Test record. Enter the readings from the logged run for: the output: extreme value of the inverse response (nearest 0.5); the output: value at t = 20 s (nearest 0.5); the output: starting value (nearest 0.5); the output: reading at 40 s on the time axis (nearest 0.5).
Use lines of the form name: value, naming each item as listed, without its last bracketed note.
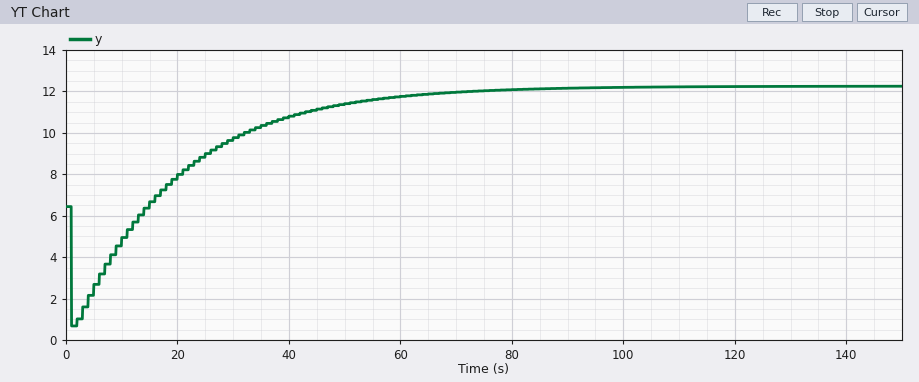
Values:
the output: extreme value of the inverse response: 0.5
the output: value at t = 20 s: 8.0
the output: starting value: 6.5
the output: reading at 40 s on the time axis: 11.0
